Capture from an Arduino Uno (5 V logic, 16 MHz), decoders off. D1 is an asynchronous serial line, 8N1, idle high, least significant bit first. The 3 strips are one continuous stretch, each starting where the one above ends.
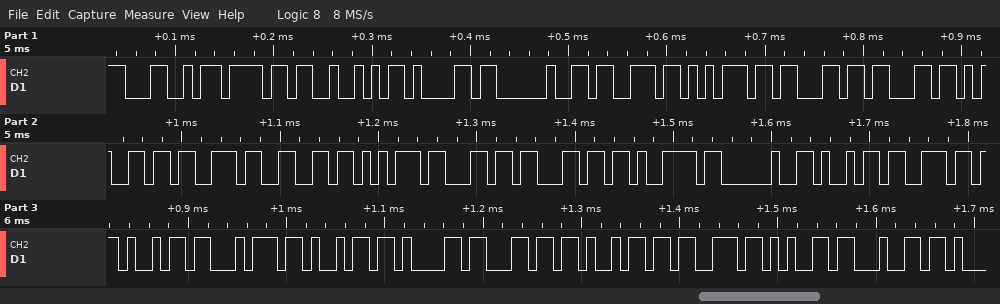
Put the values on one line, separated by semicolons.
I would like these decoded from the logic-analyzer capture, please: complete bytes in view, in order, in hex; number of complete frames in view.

4C 6F 52 61 20 73 75 63 63 65 73 66 75 6C 6C 79 20 69 6E 69 74 69 61 6C 69 73 65 64; 28
